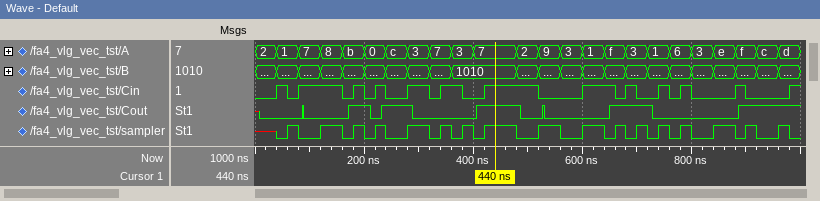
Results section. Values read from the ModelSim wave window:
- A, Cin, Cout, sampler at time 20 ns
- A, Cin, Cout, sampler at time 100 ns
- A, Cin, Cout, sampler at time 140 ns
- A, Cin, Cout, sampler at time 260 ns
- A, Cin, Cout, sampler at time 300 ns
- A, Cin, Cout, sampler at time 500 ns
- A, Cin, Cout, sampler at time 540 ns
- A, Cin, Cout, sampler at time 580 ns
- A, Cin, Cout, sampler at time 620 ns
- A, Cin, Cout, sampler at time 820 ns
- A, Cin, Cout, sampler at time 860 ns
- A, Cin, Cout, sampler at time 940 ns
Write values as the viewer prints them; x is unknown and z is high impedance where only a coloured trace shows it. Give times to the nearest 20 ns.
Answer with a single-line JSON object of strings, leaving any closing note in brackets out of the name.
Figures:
{"A, Cin, Cout, sampler at time 20 ns": "A=2, Cin=0, Cout=0, sampler=x", "A, Cin, Cout, sampler at time 100 ns": "A=7, Cin=1, Cout=0, sampler=0", "A, Cin, Cout, sampler at time 140 ns": "A=8, Cin=1, Cout=0, sampler=1", "A, Cin, Cout, sampler at time 260 ns": "A=c, Cin=0, Cout=1, sampler=0", "A, Cin, Cout, sampler at time 300 ns": "A=3, Cin=1, Cout=0, sampler=1", "A, Cin, Cout, sampler at time 500 ns": "A=2, Cin=1, Cout=0, sampler=0", "A, Cin, Cout, sampler at time 540 ns": "A=9, Cin=0, Cout=0, sampler=1", "A, Cin, Cout, sampler at time 580 ns": "A=3, Cin=0, Cout=0, sampler=0", "A, Cin, Cout, sampler at time 620 ns": "A=1, Cin=1, Cout=0, sampler=1", "A, Cin, Cout, sampler at time 820 ns": "A=3, Cin=0, Cout=0, sampler=0", "A, Cin, Cout, sampler at time 860 ns": "A=e, Cin=0, Cout=0, sampler=1", "A, Cin, Cout, sampler at time 940 ns": "A=c, Cin=0, Cout=1, sampler=0"}
